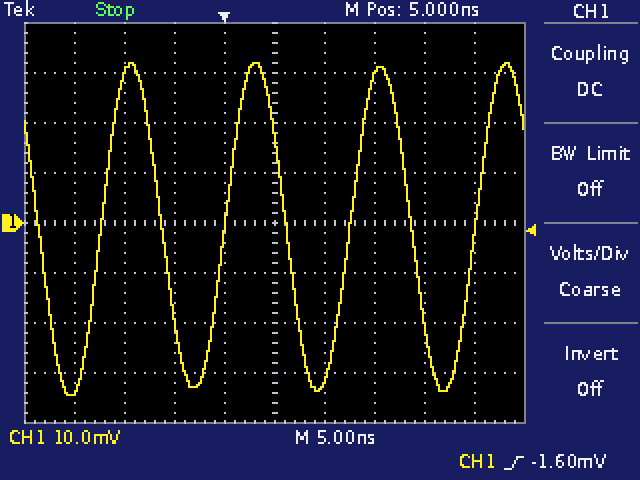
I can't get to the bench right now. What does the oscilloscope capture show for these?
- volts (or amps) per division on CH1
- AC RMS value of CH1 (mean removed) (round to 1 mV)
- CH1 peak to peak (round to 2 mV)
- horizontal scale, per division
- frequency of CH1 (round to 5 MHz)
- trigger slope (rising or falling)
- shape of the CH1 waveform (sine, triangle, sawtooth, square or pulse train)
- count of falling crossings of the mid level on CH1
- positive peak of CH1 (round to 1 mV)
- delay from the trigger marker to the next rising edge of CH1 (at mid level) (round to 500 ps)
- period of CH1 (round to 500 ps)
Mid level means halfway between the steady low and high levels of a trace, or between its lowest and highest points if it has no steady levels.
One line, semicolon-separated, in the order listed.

10 mV; 23 mV; 66 mV; 5 ns; 80 MHz; rising; sine; 4; 32 mV; 12.5 ns; 12.5 ns
